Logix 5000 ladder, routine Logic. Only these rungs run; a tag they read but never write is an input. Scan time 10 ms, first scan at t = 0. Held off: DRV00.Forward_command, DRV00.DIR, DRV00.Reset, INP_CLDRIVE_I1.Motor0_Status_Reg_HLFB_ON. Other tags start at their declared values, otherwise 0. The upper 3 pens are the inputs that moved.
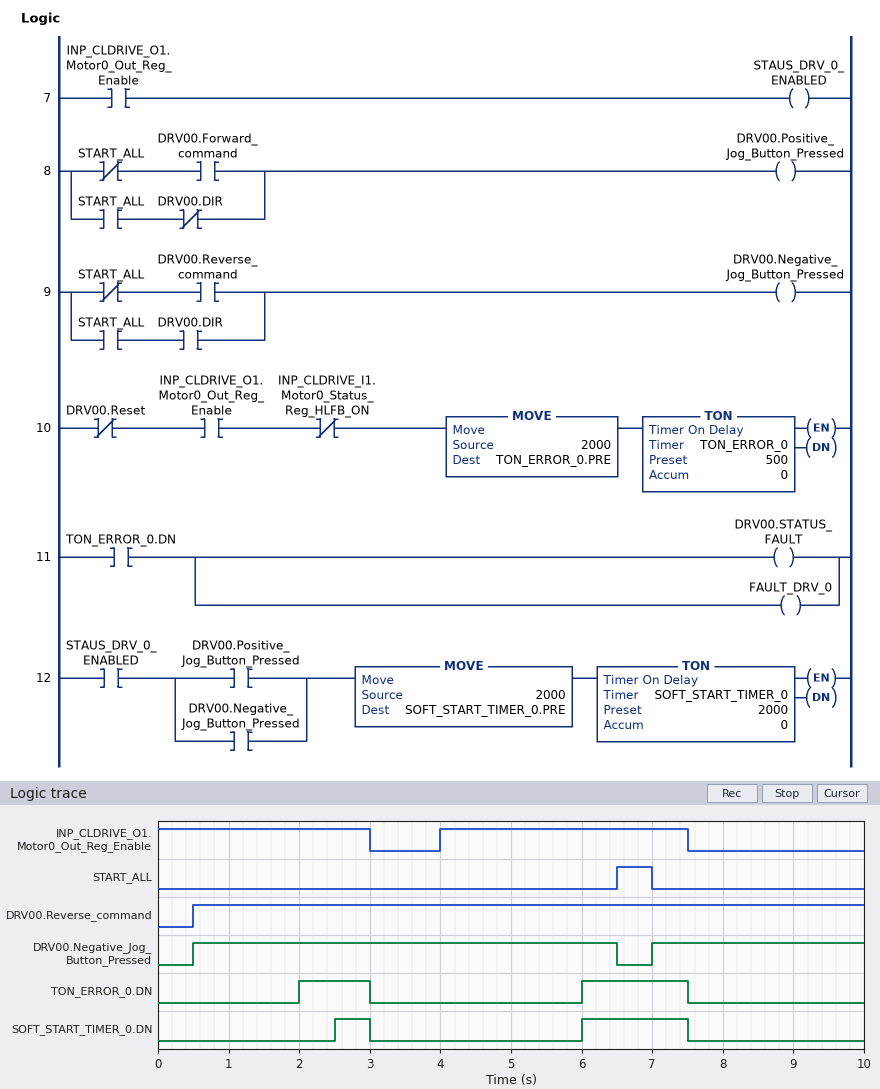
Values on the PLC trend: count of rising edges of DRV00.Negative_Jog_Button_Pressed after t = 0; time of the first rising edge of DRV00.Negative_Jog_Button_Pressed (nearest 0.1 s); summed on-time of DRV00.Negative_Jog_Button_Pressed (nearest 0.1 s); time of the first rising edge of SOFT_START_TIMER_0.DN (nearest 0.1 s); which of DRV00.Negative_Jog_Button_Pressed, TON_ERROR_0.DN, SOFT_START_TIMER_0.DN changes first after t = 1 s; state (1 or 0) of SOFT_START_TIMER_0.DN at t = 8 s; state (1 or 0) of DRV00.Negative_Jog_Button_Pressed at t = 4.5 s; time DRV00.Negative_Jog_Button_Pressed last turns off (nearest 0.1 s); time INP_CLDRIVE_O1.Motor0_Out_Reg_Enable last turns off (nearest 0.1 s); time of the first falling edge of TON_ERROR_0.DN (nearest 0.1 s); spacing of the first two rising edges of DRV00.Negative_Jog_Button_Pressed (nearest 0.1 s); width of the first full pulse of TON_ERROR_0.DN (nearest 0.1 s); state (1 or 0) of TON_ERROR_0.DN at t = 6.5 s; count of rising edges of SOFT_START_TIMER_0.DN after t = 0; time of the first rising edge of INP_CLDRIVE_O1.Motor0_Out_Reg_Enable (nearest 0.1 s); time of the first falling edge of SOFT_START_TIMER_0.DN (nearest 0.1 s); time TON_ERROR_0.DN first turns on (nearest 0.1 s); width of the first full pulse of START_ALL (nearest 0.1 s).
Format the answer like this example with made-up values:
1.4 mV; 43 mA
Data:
2; 0.5 s; 9.0 s; 2.5 s; TON_ERROR_0.DN; 0; 1; 6.5 s; 7.5 s; 3.0 s; 6.5 s; 1.0 s; 1; 2; 4.0 s; 3.0 s; 2.0 s; 0.5 s
